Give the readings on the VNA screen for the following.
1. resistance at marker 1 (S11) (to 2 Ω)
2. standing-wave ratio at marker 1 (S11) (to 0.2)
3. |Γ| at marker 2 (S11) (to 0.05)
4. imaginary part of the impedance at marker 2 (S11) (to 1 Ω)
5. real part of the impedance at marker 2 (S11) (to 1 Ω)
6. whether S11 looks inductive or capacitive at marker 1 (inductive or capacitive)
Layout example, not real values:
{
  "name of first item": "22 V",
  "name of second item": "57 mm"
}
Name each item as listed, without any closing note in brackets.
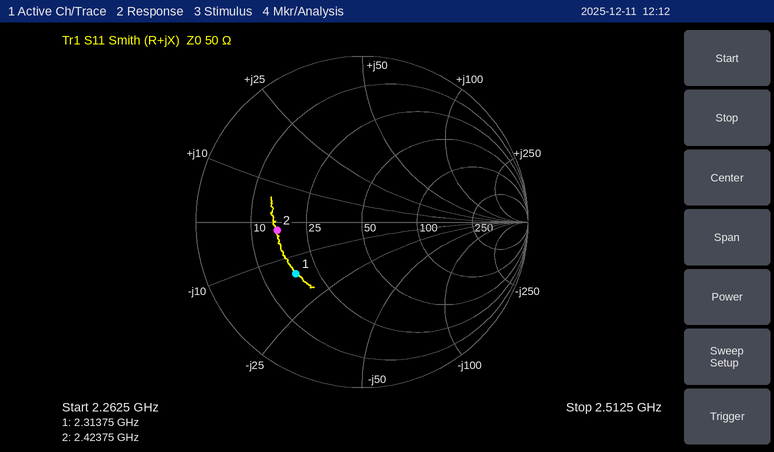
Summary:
{
  "resistance at marker 1 (S11)": "18 Ω",
  "standing-wave ratio at marker 1 (S11)": "3.0",
  "|Γ| at marker 2 (S11)": "0.50",
  "imaginary part of the impedance at marker 2 (S11)": "-2 Ω",
  "real part of the impedance at marker 2 (S11)": "16 Ω",
  "whether S11 looks inductive or capacitive at marker 1": "capacitive"
}
